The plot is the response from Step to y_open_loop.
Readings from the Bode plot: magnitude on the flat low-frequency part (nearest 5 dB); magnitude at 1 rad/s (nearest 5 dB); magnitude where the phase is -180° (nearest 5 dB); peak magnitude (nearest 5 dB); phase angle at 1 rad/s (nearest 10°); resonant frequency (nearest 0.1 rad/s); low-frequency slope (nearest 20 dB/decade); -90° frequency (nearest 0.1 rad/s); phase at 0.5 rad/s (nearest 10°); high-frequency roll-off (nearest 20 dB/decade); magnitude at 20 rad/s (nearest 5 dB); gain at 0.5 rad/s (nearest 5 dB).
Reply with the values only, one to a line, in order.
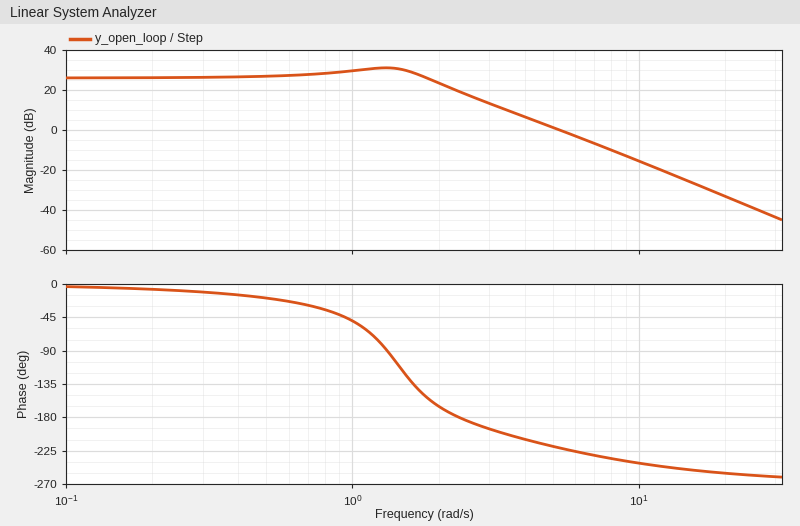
25 dB
30 dB
20 dB
30 dB
-50°
1.3 rad/s
0 dB/decade
1.3 rad/s
-20°
-60 dB/decade
-35 dB
25 dB
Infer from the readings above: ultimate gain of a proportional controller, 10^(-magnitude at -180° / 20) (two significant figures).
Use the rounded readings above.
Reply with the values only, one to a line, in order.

0.10
